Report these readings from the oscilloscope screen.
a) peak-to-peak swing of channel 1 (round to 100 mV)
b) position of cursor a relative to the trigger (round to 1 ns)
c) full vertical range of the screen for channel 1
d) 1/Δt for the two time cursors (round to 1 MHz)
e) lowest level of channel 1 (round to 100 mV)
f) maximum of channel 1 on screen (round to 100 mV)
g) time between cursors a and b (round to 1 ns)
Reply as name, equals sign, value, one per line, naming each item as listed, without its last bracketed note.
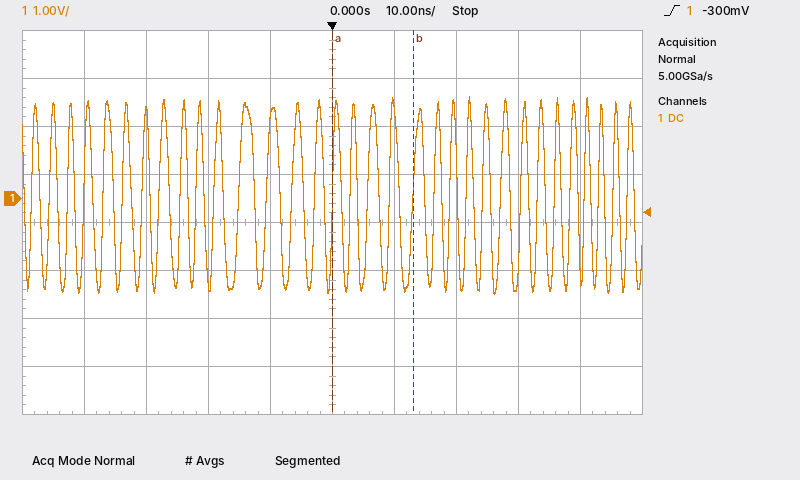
peak-to-peak swing of channel 1 = 4.1 V
position of cursor a relative to the trigger = 0 ns
full vertical range of the screen for channel 1 = 8 V
1/Δt for the two time cursors = 77 MHz
lowest level of channel 1 = -2.0 V
maximum of channel 1 on screen = 2.1 V
time between cursors a and b = 13 ns
